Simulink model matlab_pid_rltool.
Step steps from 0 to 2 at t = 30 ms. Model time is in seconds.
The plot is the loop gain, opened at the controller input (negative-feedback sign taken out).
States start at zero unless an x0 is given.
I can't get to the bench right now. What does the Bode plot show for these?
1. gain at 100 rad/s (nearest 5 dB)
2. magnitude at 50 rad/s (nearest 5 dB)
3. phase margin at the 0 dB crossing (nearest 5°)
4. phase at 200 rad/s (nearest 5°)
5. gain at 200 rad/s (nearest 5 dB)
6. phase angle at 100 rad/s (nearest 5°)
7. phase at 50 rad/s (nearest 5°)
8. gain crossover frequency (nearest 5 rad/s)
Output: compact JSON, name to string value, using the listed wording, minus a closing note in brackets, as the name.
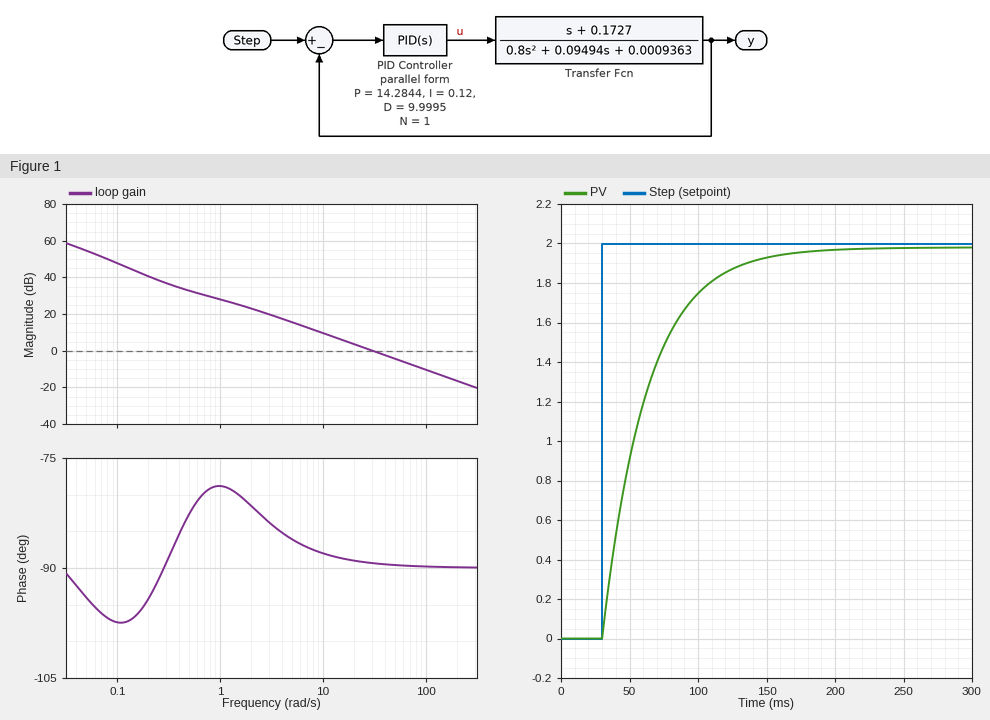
{"gain at 100 rad/s": "-10 dB", "magnitude at 50 rad/s": "-5 dB", "phase margin at the 0 dB crossing": "90°", "phase at 200 rad/s": "-90°", "gain at 200 rad/s": "-15 dB", "phase angle at 100 rad/s": "-90°", "phase at 50 rad/s": "-90°", "gain crossover frequency": "30 rad/s"}
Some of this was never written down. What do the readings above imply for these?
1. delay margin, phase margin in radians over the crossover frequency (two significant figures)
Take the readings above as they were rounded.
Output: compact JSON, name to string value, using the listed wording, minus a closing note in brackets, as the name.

{"delay margin, phase margin in radians over the crossover frequency": "0.052 s"}
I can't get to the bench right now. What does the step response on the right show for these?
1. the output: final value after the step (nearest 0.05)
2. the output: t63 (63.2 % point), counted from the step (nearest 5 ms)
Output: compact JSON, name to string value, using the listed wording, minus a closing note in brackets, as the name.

{"the output: final value after the step": "2.00", "the output: t63 (63.2 % point), counted from the step": "35 ms"}
